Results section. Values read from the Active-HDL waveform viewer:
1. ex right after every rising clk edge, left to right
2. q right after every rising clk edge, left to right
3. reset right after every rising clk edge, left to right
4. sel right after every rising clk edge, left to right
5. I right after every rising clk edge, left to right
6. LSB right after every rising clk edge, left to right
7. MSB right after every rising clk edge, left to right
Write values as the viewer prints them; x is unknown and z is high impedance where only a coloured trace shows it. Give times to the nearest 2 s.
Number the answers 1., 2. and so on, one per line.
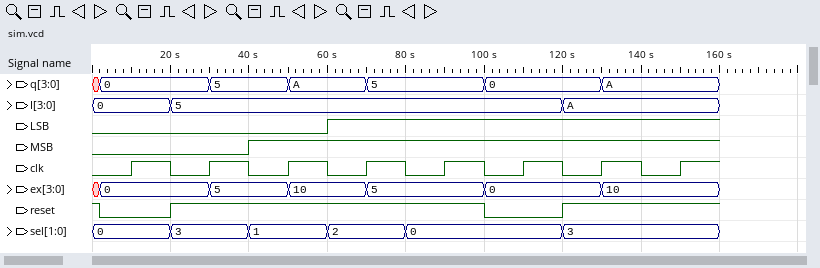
1. 0, 5, 10, 5, 5, 0, 10, 10
2. 0, 5, A, 5, 5, 0, A, A
3. 0 1 1 1 1 0 1 1
4. 0, 3, 1, 2, 0, 0, 3, 3
5. 0, 5, 5, 5, 5, 5, A, A
6. 0 0 0 1 1 1 1 1
7. 0 0 1 1 1 1 1 1
